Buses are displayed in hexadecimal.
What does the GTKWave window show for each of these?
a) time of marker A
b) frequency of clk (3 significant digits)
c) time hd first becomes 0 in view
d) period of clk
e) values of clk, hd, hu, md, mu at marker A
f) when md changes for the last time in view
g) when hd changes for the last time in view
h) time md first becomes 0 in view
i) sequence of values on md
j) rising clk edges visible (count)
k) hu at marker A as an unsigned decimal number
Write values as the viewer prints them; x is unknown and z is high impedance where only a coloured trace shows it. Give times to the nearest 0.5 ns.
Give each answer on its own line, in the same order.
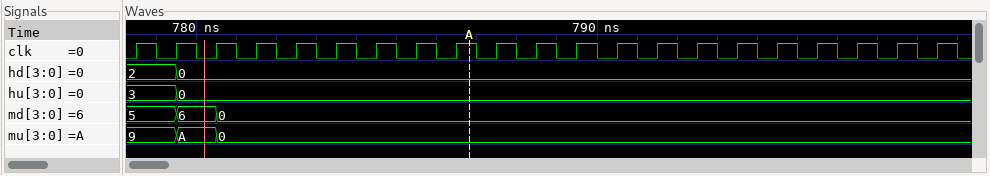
787 ns
1.00 GHz
779.5 ns
1 ns
clk=1, hd=0, hu=0, md=0, mu=0
780.5 ns
779.5 ns
780.5 ns
5, 6, 0
21
0
